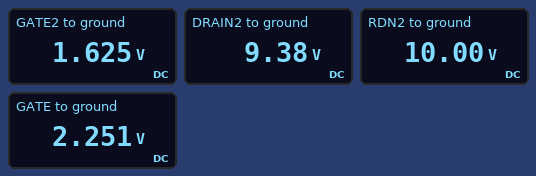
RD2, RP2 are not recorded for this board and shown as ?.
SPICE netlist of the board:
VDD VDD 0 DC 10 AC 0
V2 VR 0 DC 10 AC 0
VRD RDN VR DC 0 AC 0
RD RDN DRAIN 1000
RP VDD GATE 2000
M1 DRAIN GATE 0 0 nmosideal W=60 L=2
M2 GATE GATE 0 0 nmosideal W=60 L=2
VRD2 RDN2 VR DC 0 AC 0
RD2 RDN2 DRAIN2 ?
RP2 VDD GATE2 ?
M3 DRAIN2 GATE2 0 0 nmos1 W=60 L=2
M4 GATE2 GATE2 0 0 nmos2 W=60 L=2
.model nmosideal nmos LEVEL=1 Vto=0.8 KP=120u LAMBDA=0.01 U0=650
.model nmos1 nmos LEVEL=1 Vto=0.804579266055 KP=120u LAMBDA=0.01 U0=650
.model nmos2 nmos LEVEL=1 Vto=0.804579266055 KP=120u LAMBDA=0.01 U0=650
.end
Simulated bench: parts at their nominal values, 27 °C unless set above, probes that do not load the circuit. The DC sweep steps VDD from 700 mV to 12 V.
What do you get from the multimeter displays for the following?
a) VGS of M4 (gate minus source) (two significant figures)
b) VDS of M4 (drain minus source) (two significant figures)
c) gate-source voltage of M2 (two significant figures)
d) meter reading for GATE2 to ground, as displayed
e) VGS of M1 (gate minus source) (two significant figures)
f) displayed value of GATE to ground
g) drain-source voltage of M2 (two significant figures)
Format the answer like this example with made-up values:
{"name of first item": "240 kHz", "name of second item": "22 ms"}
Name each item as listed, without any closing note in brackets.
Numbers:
{"VGS of M4 (gate minus source)": "1.6 V", "VDS of M4 (drain minus source)": "1.6 V", "gate-source voltage of M2": "2.3 V", "meter reading for GATE2 to ground, as displayed": "1.625 V", "VGS of M1 (gate minus source)": "2.3 V", "displayed value of GATE to ground": "2.251 V", "drain-source voltage of M2": "2.3 V"}
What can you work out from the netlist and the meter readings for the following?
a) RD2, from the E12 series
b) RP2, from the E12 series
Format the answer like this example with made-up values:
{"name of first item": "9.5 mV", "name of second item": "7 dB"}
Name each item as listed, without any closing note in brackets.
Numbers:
{"RD2, from the E12 series": "470 Ω", "RP2, from the E12 series": "6.8 kΩ"}
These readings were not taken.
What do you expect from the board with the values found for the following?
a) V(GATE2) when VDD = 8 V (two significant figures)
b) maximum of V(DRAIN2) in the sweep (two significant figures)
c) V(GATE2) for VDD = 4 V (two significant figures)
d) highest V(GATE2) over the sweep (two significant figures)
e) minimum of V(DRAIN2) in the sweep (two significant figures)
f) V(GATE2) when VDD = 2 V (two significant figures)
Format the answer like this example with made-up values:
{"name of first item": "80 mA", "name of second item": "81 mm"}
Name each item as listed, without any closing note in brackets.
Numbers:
{"V(GATE2) when VDD = 8 V": "1.5 V", "maximum of V(DRAIN2) in the sweep": "10 V", "V(GATE2) for VDD = 4 V": "1.3 V", "highest V(GATE2) over the sweep": "1.7 V", "minimum of V(DRAIN2) in the sweep": "9.2 V", "V(GATE2) when VDD = 2 V": "1.1 V"}
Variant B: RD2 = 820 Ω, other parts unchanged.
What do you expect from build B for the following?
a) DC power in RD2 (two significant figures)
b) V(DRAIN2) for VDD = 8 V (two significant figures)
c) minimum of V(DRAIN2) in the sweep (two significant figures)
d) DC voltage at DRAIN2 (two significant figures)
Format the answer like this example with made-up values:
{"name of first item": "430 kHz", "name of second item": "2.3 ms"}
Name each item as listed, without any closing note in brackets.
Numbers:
{"DC power in RD2": "1.4 mW", "V(DRAIN2) for VDD = 8 V": "9.2 V", "minimum of V(DRAIN2) in the sweep": "8.7 V", "DC voltage at DRAIN2": "8.9 V"}
